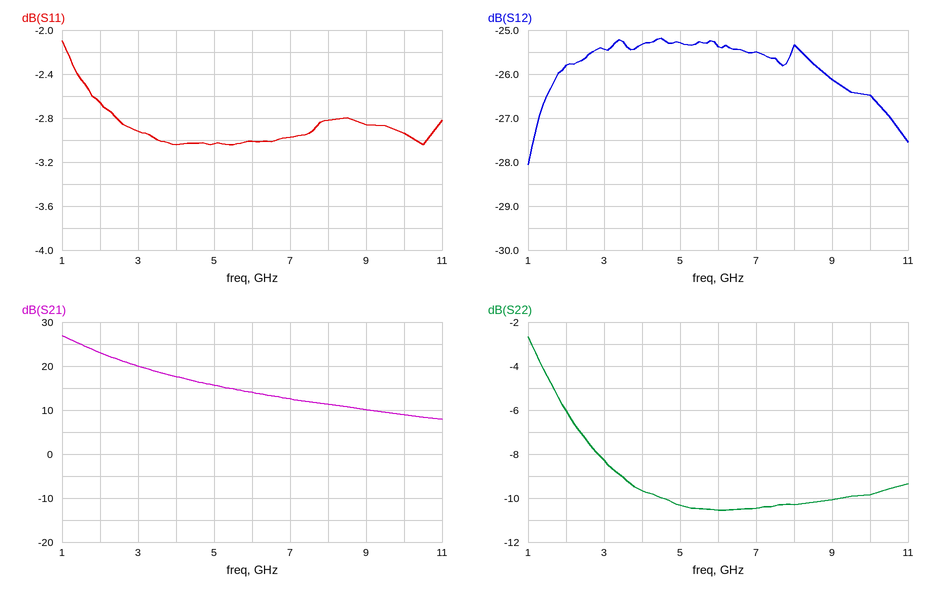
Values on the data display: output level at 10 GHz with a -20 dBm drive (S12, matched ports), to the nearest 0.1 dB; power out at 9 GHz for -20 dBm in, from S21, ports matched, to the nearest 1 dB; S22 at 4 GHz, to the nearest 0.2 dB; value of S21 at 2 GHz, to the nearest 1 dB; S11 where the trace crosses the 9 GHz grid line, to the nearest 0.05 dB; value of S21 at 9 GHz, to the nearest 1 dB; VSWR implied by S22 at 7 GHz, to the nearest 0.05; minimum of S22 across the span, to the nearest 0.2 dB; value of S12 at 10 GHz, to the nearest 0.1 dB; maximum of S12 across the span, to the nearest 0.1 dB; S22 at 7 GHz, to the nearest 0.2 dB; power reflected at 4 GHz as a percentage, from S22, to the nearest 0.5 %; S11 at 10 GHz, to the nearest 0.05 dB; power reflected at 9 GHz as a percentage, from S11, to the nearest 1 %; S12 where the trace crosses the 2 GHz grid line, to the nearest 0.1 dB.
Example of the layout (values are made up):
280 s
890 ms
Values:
-46.5 dBm
-10 dBm
-9.6 dB
23 dB
-2.85 dB
10 dB
1.85
-10.6 dB
-26.5 dB
-25.2 dB
-10.4 dB
11.0 %
-2.95 dB
52 %
-25.8 dB
